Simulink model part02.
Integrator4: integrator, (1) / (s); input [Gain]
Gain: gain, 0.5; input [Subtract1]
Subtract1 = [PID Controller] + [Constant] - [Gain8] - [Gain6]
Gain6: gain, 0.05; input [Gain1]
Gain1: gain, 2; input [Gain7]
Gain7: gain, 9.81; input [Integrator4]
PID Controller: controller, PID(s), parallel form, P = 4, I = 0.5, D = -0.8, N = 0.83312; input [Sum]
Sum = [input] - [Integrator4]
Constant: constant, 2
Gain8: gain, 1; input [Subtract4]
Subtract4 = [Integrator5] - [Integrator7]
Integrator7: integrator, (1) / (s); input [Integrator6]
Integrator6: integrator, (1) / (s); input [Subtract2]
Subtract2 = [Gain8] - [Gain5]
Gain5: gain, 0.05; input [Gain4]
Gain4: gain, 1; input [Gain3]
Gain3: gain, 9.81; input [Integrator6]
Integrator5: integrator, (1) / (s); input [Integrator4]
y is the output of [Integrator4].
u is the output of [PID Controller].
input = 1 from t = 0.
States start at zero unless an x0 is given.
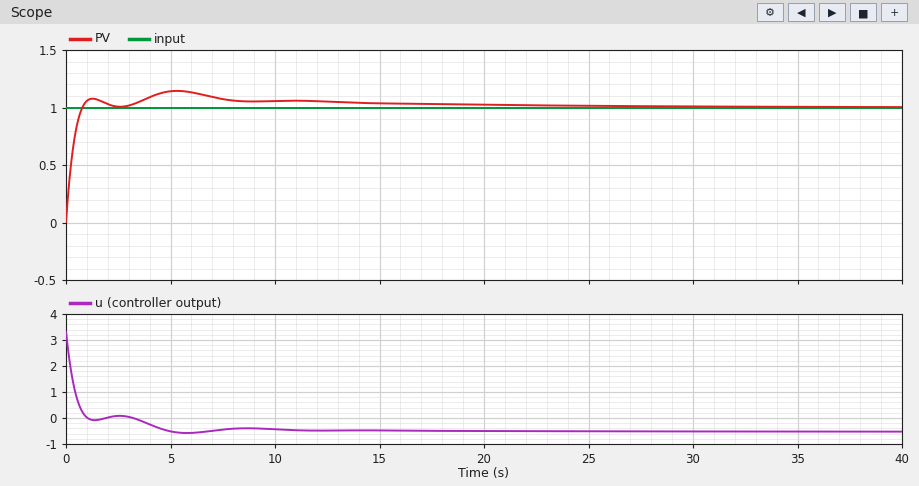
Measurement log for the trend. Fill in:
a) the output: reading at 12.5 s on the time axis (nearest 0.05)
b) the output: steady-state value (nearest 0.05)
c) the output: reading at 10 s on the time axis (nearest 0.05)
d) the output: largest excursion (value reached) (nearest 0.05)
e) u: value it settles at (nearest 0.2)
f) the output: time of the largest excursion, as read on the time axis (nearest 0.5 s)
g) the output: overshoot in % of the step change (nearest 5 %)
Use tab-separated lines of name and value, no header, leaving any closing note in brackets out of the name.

the output: reading at 12.5 s on the time axis	1.05
the output: steady-state value	1.00
the output: reading at 10 s on the time axis	1.05
the output: largest excursion (value reached)	1.15
u: value it settles at	-0.6
the output: time of the largest excursion, as read on the time axis	5.5 s
the output: overshoot in % of the step change	15 %
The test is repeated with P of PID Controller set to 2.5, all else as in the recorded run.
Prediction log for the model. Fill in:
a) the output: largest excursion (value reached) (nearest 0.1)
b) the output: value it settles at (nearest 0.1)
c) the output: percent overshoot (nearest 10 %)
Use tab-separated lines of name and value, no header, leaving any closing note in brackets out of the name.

the output: largest excursion (value reached)	1.2
the output: value it settles at	1.0
the output: percent overshoot	20 %
